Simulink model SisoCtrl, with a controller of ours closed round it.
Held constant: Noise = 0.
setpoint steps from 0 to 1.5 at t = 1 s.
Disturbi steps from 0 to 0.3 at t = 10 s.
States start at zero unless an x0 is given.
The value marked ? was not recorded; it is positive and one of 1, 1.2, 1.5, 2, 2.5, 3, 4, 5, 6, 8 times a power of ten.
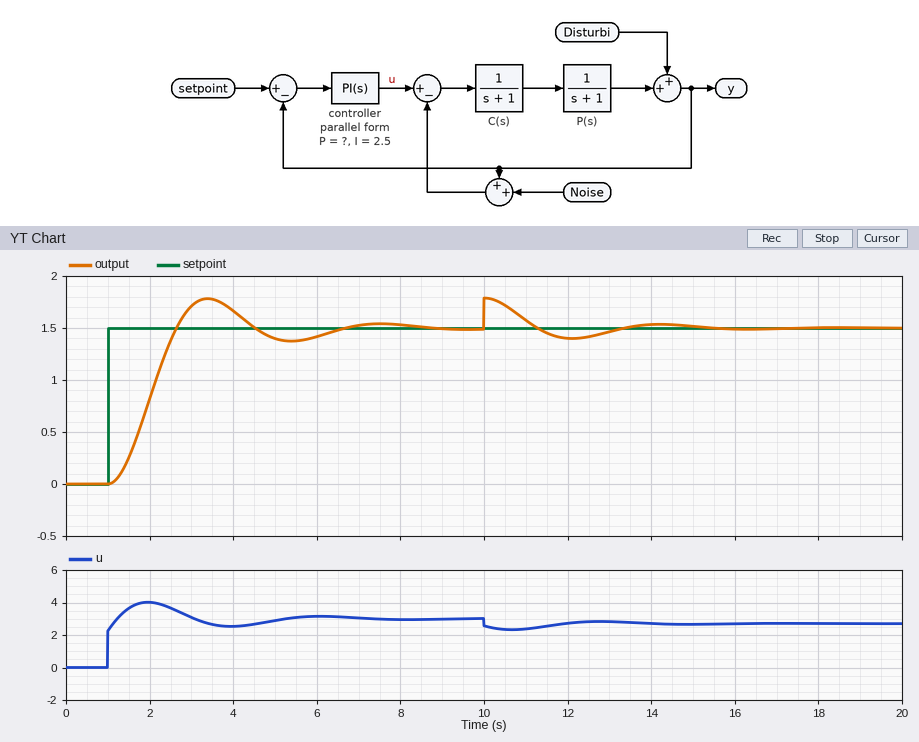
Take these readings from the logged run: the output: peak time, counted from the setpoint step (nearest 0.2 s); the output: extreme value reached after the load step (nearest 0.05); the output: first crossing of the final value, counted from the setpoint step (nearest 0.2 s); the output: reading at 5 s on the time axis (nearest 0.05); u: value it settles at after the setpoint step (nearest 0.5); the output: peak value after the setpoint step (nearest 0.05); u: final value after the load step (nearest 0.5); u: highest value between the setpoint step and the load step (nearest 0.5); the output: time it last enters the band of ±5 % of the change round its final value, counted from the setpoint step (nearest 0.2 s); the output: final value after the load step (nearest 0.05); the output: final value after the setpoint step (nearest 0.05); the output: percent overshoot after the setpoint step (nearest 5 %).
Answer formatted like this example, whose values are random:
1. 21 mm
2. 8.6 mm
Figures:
1. 2.4 s
2. 1.80
3. 1.6 s
4. 1.40
5. 3.0
6. 1.80
7. 2.5
8. 4.0
9. 5.0 s
10. 1.50
11. 1.50
12. 20 %
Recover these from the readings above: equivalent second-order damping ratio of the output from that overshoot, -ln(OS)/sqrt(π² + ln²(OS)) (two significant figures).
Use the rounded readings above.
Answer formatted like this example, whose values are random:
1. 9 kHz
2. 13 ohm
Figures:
1. 0.46
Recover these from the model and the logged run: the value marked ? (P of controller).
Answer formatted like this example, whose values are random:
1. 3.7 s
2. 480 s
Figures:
1. 1.5
